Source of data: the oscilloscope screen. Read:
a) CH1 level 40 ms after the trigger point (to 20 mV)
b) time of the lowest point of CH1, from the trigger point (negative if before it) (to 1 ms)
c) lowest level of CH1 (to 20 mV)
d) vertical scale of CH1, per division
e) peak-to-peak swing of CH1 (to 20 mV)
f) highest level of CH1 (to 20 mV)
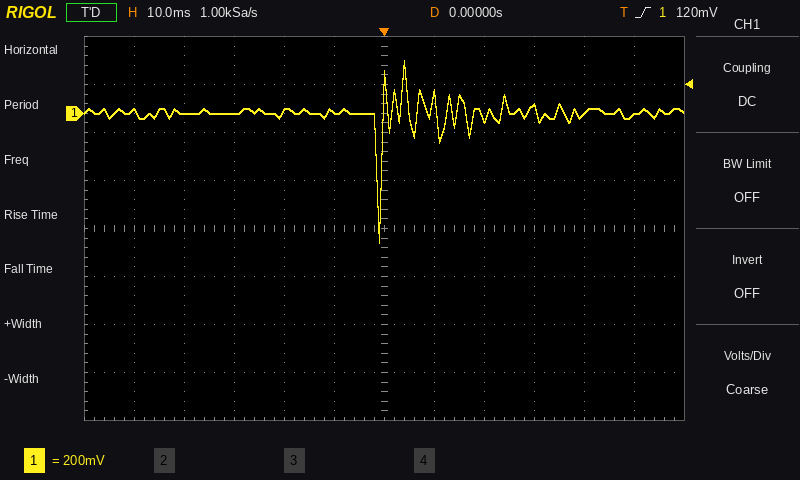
0 mV
-1 ms
-540 mV
200 mV
760 mV
220 mV
